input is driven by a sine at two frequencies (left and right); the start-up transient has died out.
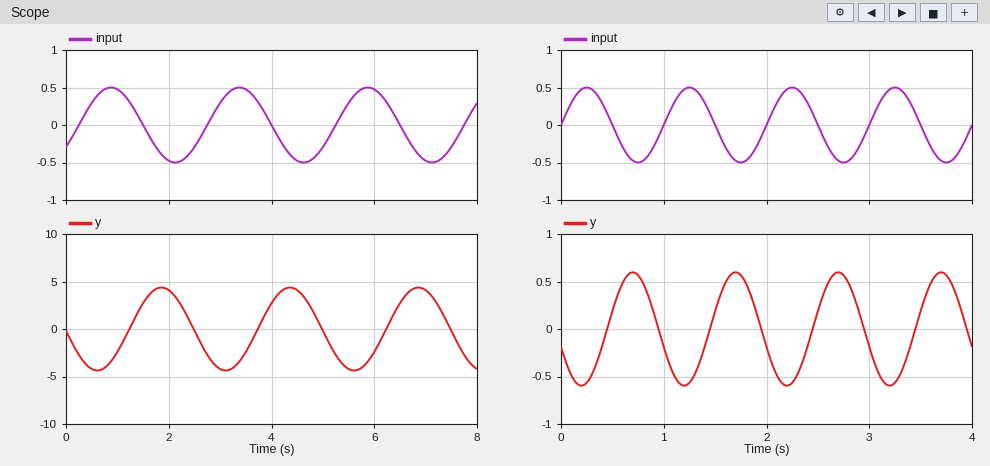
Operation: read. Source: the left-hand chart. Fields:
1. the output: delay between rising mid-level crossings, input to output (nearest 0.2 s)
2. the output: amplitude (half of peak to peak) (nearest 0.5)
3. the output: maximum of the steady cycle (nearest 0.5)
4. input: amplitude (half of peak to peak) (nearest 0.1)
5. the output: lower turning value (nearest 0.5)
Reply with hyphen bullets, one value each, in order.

- 1.0 s
- 4.5
- 4.5
- 0.5
- -4.5
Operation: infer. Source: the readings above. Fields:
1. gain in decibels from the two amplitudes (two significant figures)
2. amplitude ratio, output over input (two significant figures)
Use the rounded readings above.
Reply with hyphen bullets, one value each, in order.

- 19 dB
- 9.0
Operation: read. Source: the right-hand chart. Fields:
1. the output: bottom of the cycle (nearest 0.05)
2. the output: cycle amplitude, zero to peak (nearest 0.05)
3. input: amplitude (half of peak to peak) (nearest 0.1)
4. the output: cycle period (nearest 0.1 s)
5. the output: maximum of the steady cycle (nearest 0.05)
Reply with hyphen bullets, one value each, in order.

- -0.60
- 0.60
- 0.5
- 1.0 s
- 0.60
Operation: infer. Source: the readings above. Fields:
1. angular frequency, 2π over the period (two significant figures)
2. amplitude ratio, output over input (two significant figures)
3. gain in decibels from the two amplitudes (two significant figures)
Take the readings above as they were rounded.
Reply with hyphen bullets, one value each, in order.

- 6.3 rad/s
- 1.2
- 1.6 dB
